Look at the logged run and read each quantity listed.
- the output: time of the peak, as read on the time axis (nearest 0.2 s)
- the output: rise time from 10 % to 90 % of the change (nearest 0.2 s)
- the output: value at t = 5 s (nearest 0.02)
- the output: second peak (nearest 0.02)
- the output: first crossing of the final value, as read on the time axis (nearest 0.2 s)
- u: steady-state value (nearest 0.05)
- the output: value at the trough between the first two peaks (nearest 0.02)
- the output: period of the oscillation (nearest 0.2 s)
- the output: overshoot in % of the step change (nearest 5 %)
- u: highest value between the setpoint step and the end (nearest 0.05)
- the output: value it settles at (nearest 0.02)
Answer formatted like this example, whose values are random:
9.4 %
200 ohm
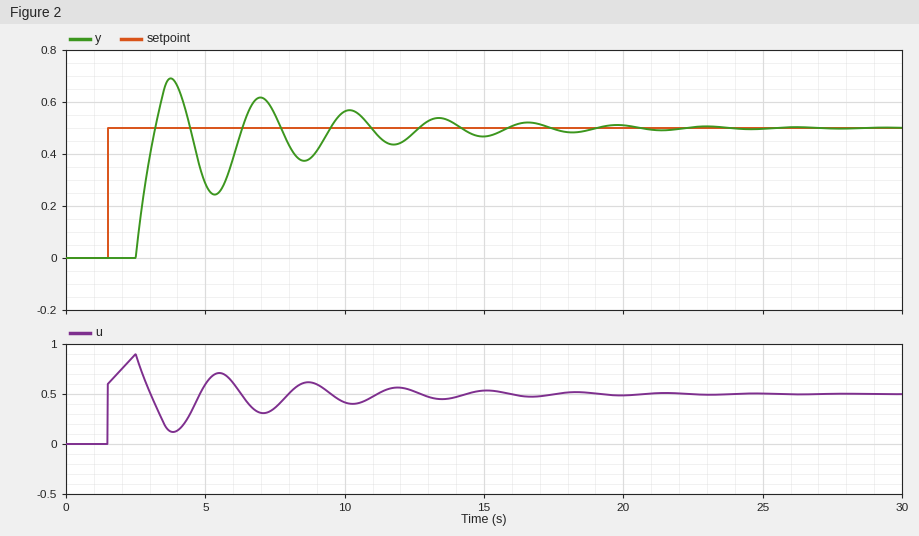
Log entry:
3.8 s
0.6 s
0.28
0.62
3.2 s
0.50
0.24
3.2 s
40 %
0.90
0.50
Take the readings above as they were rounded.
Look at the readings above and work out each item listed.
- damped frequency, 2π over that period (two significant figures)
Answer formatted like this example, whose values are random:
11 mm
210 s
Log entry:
2.0 rad/s
